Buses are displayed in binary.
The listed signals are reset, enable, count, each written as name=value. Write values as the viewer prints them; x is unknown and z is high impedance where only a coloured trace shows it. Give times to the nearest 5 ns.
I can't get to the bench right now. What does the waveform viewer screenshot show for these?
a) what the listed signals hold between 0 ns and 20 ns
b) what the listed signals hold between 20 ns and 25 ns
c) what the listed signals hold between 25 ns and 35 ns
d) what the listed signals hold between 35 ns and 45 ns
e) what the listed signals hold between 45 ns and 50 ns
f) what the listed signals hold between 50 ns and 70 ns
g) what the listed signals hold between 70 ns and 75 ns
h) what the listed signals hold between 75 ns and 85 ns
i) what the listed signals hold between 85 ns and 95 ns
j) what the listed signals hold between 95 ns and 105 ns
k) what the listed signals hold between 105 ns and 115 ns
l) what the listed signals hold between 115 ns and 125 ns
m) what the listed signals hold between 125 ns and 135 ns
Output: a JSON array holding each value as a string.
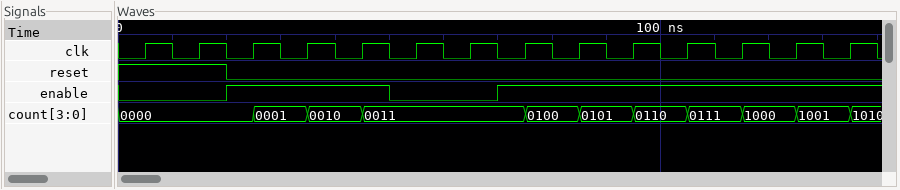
["reset=1, enable=0, count=0000", "reset=0, enable=1, count=0000", "reset=0, enable=1, count=0001", "reset=0, enable=1, count=0010", "reset=0, enable=1, count=0011", "reset=0, enable=0, count=0011", "reset=0, enable=1, count=0011", "reset=0, enable=1, count=0100", "reset=0, enable=1, count=0101", "reset=0, enable=1, count=0110", "reset=0, enable=1, count=0111", "reset=0, enable=1, count=1000", "reset=0, enable=1, count=1001"]
